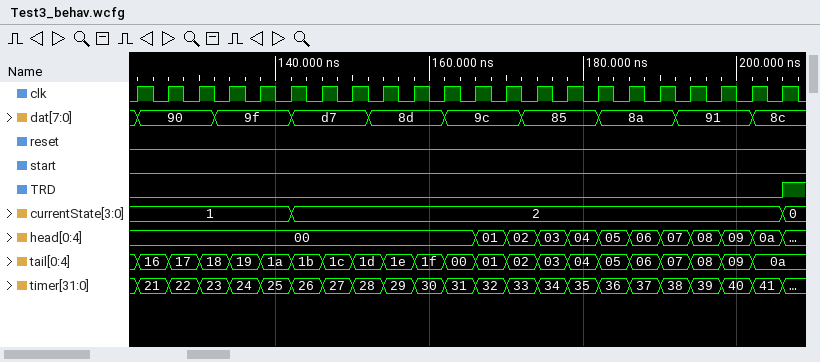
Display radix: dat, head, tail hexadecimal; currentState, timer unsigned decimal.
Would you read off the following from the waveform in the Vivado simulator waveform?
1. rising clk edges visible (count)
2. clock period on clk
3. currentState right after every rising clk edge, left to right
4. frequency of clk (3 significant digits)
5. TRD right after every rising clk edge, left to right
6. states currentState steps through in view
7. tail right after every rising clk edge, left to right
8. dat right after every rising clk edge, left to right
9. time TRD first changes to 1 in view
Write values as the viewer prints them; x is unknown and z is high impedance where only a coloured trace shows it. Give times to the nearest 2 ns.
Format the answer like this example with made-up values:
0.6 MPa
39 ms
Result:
22
4 ns
1, 1, 1, 1, 1, 2, 2, 2, 2, 2, 2, 2, 2, 2, 2, 2, 2, 2, 2, 2, 2, 0
250 MHz
0 0 0 0 0 0 0 0 0 0 0 0 0 0 0 0 0 0 0 0 0 1
1, 2, 0
16, 17, 18, 19, 1a, 1b, 1c, 1d, 1e, 1f, 00, 01, 02, 03, 04, 05, 06, 07, 08, 09, 0a, 0a
90, 90, 90, 9f, 9f, d7, d7, d7, 8d, 8d, 9c, 9c, 9c, 85, 85, 8a, 8a, 8a, 91, 91, 8c, 8c
206 ns
